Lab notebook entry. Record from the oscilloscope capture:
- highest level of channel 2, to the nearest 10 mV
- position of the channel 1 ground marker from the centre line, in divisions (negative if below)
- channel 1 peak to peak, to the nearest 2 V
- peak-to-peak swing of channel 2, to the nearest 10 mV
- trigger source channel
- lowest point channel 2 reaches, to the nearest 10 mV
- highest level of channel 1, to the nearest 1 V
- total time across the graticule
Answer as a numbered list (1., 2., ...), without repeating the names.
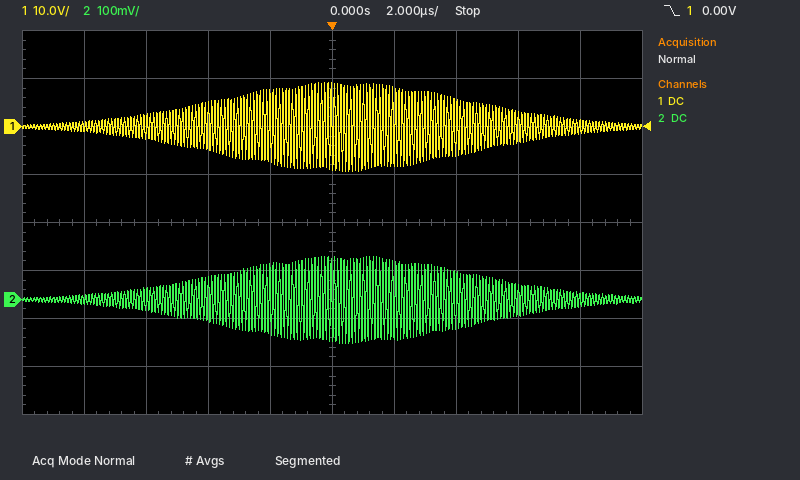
1. 90 mV
2. +2.0 div
3. 18 V
4. 180 mV
5. channel 1
6. -90 mV
7. 9 V
8. 20 µs
